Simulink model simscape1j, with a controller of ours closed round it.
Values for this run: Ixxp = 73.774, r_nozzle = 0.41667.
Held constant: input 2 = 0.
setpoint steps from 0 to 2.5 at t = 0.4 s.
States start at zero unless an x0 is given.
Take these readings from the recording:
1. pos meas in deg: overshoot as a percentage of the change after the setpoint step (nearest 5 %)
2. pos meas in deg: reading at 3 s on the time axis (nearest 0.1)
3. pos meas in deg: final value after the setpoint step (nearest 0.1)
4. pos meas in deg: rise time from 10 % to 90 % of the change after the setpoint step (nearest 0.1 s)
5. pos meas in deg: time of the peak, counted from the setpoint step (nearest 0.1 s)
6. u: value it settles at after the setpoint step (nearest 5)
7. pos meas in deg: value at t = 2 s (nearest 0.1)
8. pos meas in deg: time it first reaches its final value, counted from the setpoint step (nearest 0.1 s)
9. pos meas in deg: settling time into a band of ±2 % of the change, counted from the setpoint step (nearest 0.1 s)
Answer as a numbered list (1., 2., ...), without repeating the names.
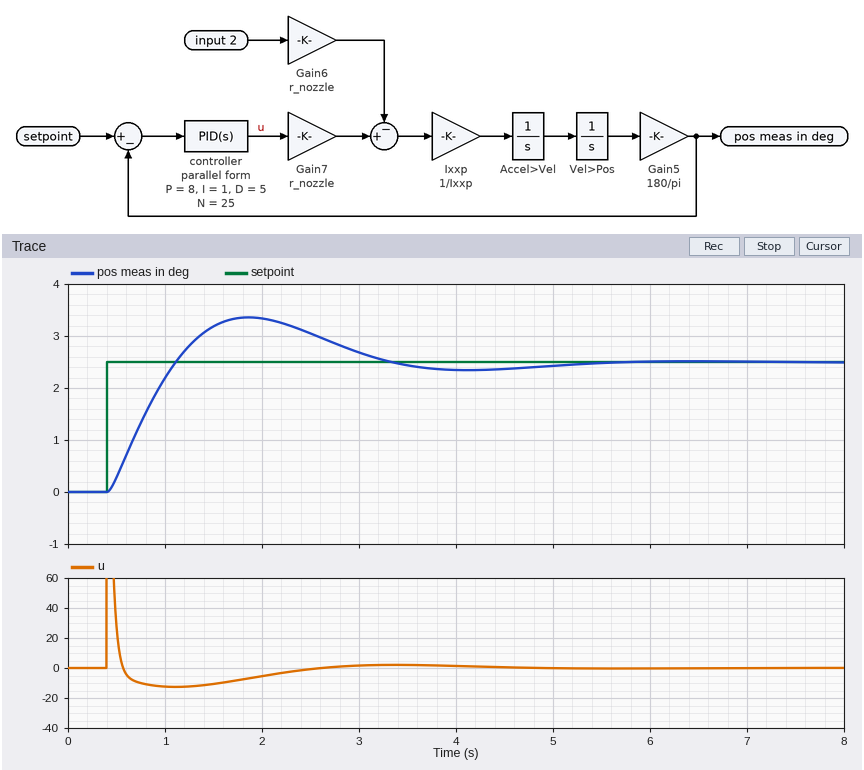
1. 35 %
2. 2.7
3. 2.5
4. 0.5 s
5. 1.5 s
6. 0
7. 3.3
8. 0.7 s
9. 4.8 s
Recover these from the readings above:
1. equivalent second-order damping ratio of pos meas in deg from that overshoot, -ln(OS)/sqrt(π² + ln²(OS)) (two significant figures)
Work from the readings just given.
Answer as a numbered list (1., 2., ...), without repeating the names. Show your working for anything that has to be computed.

1. ln(0.35) = -1.050; 1.050 / sqrt(9.870 + 1.102) = 0.32
